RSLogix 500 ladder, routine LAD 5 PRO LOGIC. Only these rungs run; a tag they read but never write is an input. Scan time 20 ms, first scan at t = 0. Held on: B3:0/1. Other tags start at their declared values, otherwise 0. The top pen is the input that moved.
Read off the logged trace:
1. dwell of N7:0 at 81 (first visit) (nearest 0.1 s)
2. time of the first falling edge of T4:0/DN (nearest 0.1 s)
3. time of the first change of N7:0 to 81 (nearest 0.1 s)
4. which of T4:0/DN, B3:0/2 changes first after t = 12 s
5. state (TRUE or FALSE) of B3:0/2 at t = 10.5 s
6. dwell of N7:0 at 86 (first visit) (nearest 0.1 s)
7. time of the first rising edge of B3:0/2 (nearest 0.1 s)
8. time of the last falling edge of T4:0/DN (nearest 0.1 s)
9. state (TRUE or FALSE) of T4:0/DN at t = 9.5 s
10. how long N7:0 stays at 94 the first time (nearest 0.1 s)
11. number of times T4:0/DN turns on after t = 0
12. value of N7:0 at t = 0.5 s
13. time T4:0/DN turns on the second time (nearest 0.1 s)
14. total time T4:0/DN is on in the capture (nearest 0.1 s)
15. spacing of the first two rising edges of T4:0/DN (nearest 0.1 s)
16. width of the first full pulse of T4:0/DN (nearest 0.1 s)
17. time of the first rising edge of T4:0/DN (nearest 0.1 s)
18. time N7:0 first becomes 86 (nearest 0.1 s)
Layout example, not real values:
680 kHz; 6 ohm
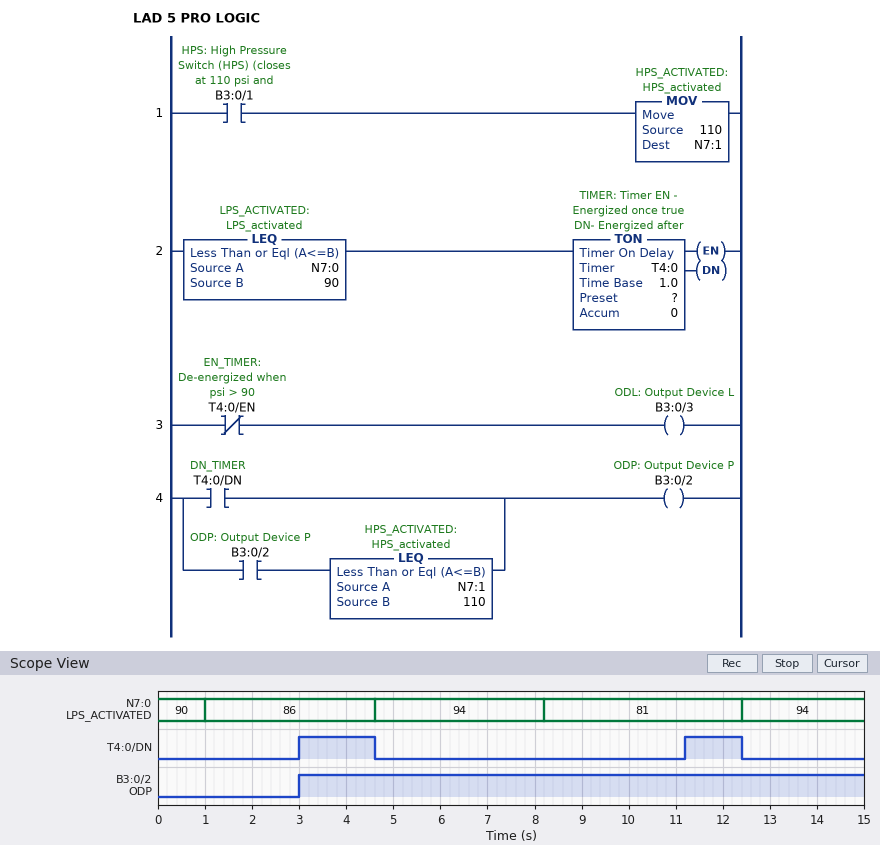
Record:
4.2 s; 4.6 s; 8.2 s; T4:0/DN; TRUE; 3.6 s; 3.0 s; 12.4 s; FALSE; 3.6 s; 2; 90; 11.2 s; 2.8 s; 8.2 s; 1.6 s; 3.0 s; 1.0 s
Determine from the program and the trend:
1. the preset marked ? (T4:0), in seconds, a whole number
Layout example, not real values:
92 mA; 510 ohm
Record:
3 s
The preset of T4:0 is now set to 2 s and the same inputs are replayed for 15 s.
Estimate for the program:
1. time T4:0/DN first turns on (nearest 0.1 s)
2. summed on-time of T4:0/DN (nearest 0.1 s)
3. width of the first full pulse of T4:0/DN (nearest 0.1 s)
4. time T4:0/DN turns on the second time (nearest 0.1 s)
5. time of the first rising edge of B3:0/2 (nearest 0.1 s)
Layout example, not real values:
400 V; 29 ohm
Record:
2.0 s; 4.8 s; 2.6 s; 10.2 s; 2.0 s
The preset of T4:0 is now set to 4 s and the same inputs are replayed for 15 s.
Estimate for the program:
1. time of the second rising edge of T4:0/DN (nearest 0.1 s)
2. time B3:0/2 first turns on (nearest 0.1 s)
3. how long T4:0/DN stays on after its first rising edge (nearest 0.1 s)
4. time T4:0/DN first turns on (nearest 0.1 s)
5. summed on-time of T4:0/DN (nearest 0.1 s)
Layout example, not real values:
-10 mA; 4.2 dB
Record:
12.2 s; 4.0 s; 0.6 s; 4.0 s; 0.8 s
